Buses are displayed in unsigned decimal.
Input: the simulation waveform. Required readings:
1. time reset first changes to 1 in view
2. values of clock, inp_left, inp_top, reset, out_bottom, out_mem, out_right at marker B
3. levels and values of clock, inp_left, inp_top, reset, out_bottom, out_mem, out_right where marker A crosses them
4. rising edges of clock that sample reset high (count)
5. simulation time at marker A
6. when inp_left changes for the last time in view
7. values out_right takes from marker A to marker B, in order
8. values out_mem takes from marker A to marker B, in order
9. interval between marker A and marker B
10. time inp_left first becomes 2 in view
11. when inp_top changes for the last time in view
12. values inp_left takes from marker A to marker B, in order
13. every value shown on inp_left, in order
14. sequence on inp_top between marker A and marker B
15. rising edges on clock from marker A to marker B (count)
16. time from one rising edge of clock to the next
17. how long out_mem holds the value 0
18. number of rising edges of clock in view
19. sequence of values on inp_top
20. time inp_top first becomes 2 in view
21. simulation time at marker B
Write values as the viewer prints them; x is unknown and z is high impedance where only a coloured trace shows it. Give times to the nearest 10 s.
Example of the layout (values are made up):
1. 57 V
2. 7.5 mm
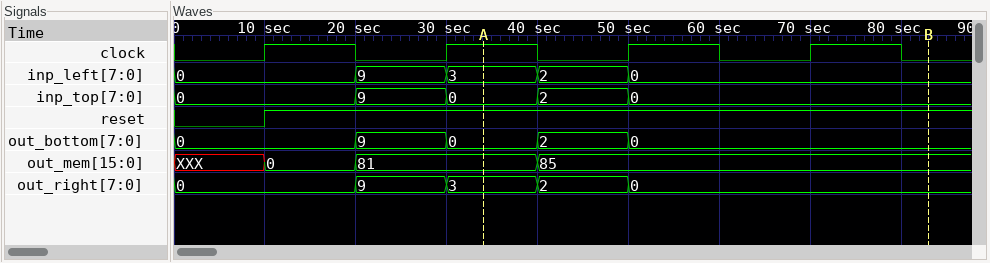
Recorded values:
1. 10 s
2. clock=0, inp_left=0, inp_top=0, reset=1, out_bottom=0, out_mem=85, out_right=0
3. clock=1, inp_left=3, inp_top=0, reset=1, out_bottom=0, out_mem=81, out_right=3
4. 3
5. 30 s
6. 50 s
7. 3, 2, 0
8. 81, 85
9. 50 s
10. 40 s
11. 50 s
12. 3, 2, 0
13. 0, 9, 3, 2, 0
14. 0, 2, 0
15. 2
16. 20 s
17. 10 s
18. 4
19. 0, 9, 0, 2, 0
20. 40 s
21. 80 s
